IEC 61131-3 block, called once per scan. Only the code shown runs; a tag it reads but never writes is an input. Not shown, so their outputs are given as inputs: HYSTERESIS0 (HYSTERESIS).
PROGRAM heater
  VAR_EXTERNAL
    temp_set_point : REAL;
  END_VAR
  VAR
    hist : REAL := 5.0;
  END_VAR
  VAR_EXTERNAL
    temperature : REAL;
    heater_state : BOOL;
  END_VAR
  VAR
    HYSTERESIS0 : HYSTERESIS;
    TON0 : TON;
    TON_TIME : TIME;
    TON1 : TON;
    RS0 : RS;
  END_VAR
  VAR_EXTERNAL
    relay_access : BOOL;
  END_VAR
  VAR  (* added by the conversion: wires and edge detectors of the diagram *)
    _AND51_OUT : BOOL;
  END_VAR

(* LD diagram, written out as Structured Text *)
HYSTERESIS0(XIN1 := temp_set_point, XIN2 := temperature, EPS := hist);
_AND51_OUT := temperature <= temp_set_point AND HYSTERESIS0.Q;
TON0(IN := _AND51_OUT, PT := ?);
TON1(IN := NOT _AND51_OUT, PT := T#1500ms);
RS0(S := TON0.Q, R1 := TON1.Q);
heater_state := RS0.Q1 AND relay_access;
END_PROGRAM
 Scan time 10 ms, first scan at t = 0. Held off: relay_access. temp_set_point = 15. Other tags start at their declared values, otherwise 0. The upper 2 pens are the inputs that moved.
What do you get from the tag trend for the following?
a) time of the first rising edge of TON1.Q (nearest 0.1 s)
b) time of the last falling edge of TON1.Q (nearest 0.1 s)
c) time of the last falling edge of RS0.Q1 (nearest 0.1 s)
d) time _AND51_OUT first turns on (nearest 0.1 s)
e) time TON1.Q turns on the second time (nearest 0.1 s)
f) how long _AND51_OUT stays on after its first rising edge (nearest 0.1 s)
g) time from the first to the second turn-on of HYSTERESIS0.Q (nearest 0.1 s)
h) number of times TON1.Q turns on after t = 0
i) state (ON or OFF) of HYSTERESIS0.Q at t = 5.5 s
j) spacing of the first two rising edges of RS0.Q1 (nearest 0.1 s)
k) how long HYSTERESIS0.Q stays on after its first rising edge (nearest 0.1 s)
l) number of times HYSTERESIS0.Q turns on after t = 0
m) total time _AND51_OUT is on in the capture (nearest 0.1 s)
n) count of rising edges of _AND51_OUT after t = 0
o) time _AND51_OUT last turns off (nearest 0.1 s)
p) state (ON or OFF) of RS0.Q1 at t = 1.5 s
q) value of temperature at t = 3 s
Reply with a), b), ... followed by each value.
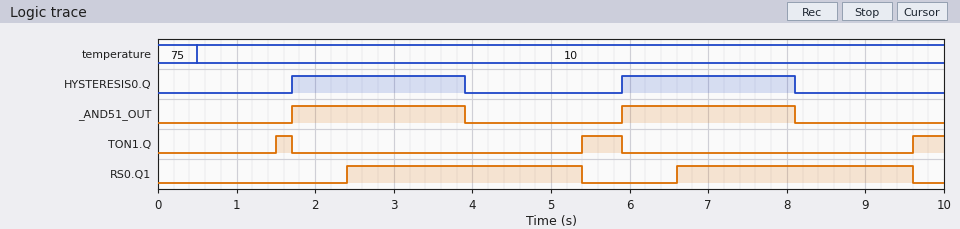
a) 1.5 s
b) 5.9 s
c) 9.6 s
d) 1.7 s
e) 5.4 s
f) 2.2 s
g) 4.2 s
h) 3
i) OFF
j) 4.2 s
k) 2.2 s
l) 2
m) 4.4 s
n) 2
o) 8.1 s
p) OFF
q) 10
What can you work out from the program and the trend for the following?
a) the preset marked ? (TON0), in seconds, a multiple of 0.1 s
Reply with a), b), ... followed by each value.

a) 0.7 s
